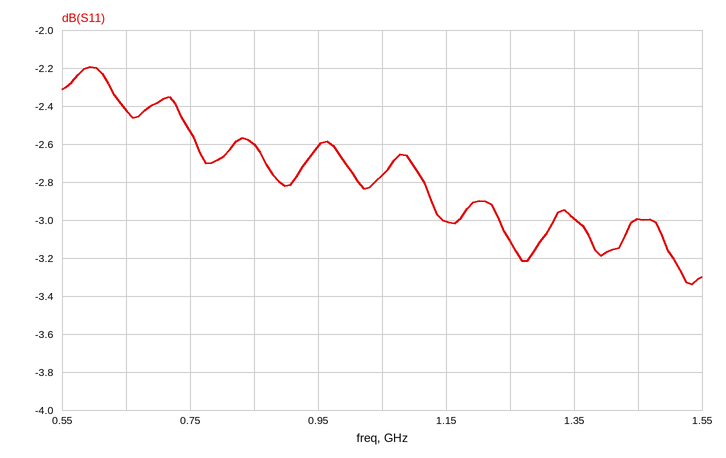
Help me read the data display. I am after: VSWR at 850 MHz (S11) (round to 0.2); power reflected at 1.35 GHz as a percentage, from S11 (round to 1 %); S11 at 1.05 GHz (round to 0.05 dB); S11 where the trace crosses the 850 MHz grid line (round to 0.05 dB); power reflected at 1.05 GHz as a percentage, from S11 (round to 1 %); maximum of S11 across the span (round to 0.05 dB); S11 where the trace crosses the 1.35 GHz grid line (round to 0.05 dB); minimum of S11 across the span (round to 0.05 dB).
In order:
6.8
50 %
-2.75 dB
-2.60 dB
53 %
-2.20 dB
-3.00 dB
-3.35 dB
